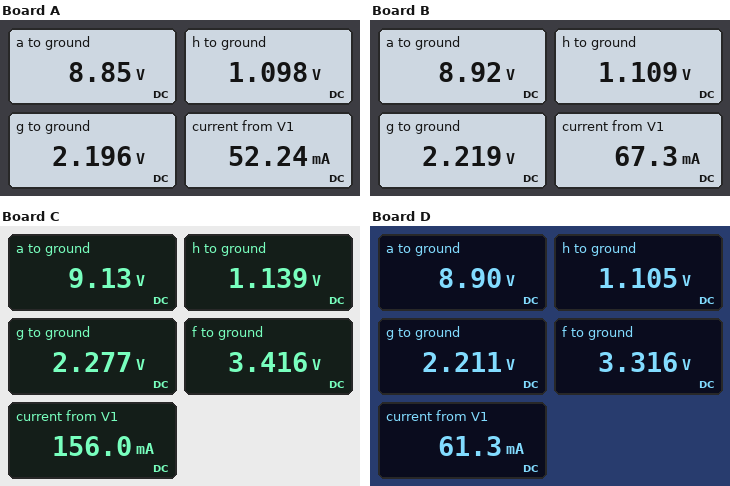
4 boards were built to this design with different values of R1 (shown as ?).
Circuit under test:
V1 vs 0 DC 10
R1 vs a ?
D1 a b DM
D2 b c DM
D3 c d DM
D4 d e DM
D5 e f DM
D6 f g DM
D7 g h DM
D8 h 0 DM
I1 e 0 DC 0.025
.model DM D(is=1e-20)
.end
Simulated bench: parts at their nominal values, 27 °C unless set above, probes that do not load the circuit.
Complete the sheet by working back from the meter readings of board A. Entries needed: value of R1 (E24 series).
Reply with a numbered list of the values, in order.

1. 22 Ω
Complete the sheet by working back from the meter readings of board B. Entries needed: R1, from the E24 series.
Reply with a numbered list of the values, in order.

1. 16 Ω
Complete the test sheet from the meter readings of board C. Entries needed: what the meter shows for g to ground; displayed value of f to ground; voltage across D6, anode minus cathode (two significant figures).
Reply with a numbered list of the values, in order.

1. 2.277 V
2. 3.416 V
3. 1.1 V
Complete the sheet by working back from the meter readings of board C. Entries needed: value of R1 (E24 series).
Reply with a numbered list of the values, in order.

1. 5.6 Ω
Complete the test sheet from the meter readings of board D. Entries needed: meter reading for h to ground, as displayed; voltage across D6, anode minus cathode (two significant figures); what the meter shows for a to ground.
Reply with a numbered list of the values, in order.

1. 1.105 V
2. 1.1 V
3. 8.90 V
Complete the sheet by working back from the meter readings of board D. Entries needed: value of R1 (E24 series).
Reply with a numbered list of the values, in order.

1. 18 Ω
